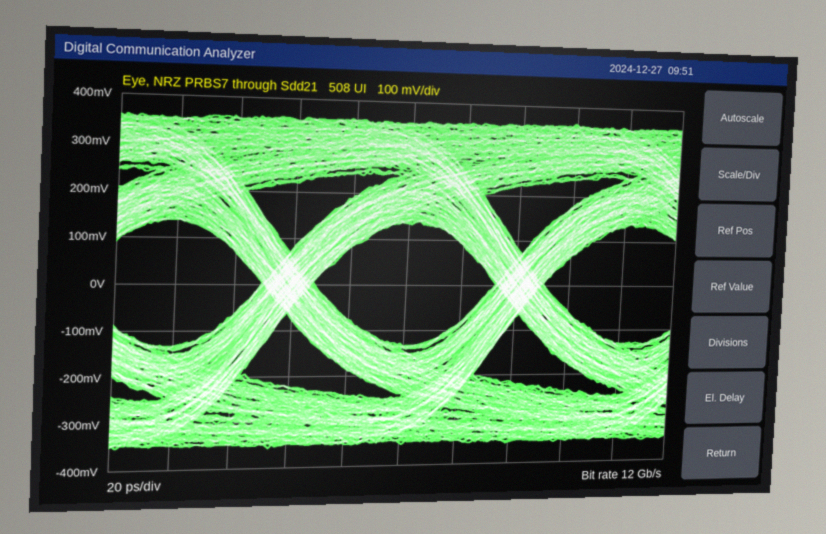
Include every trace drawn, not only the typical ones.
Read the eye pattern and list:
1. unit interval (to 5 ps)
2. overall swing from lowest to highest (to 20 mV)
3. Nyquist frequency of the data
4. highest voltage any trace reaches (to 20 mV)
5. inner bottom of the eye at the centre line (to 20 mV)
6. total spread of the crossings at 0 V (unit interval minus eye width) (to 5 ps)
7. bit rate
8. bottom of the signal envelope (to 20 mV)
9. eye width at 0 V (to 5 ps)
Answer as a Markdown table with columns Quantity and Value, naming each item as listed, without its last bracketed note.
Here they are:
| Quantity | Value |
|---|---|
| unit interval | 85 ps |
| overall swing from lowest to highest | 720 mV |
| Nyquist frequency of the data | 6 GHz |
| highest voltage any trace reaches | 360 mV |
| inner bottom of the eye at the centre line | -140 mV |
| total spread of the crossings at 0 V (unit interval minus eye width) | 20 ps |
| bit rate | 12 Gb/s |
| bottom of the signal envelope | -360 mV |
| eye width at 0 V | 65 ps |
